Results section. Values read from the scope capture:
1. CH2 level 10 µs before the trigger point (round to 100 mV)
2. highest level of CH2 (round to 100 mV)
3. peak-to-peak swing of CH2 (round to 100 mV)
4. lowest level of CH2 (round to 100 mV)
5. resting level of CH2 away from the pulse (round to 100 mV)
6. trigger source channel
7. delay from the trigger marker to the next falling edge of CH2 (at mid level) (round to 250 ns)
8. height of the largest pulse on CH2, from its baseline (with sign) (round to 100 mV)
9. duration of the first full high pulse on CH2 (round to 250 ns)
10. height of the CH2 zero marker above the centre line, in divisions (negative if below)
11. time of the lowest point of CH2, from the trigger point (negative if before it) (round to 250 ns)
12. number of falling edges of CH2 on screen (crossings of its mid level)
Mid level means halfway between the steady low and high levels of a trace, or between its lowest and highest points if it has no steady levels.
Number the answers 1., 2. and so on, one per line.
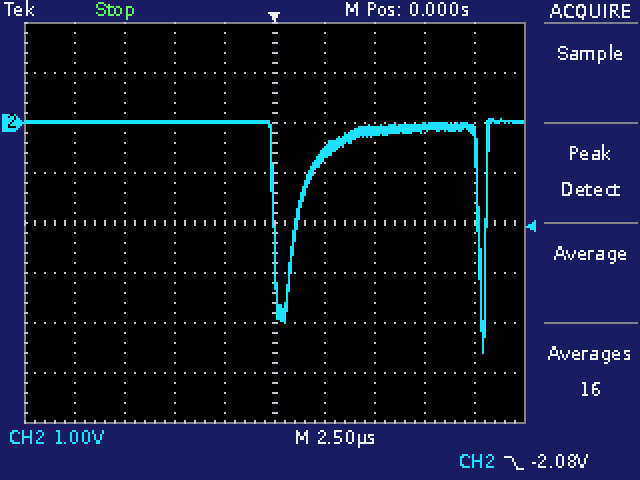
1. 0.0 V
2. 100 mV
3. 4.7 V
4. -4.6 V
5. 0.0 V
6. CH2
7. 10.25 µs
8. -4.6 V
9. 9.25 µs
10. +2.0 div
11. +10.50 µs
12. 2
